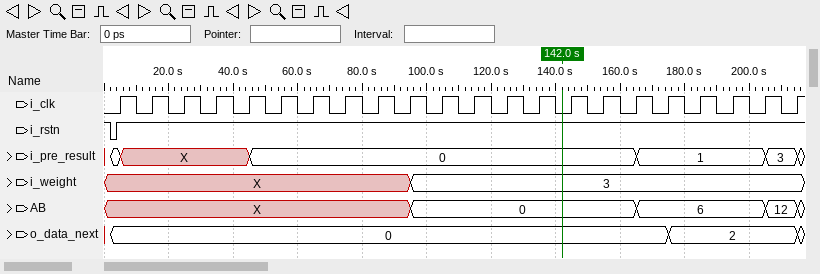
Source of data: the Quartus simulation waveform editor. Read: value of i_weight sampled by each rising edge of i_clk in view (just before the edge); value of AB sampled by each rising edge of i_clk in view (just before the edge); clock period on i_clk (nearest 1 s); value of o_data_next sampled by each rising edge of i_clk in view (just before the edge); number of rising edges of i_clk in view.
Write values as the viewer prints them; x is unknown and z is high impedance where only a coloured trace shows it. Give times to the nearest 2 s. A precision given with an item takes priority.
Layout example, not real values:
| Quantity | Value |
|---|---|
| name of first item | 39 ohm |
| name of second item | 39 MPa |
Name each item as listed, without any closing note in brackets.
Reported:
| Quantity | Value |
|---|---|
| value of i_weight sampled by each rising edge of i_clk in view | X, X, X, X, X, X, X, X, X, X, 3, 3, 3, 3, 3, 3, 3, 3, 3, 3, 3, 3 |
| value of AB sampled by each rising edge of i_clk in view | X, X, X, X, X, X, X, X, X, X, 0, 0, 0, 0, 0, 0, 0, 6, 6, 6, 6, 12 |
| clock period on i_clk | 10 s |
| value of o_data_next sampled by each rising edge of i_clk in view | 0, 0, 0, 0, 0, 0, 0, 0, 0, 0, 0, 0, 0, 0, 0, 0, 0, 0, 2, 2, 2, 2 |
| number of rising edges of i_clk in view | 22 |
